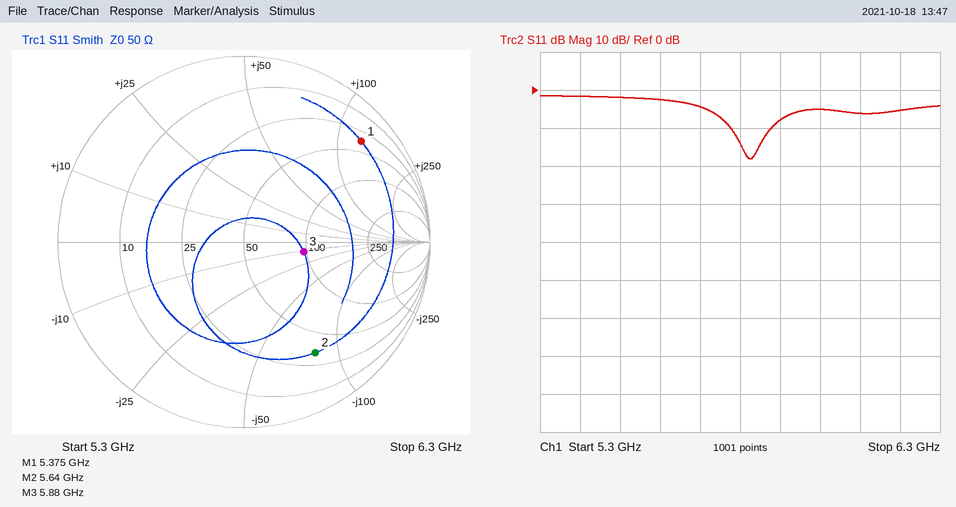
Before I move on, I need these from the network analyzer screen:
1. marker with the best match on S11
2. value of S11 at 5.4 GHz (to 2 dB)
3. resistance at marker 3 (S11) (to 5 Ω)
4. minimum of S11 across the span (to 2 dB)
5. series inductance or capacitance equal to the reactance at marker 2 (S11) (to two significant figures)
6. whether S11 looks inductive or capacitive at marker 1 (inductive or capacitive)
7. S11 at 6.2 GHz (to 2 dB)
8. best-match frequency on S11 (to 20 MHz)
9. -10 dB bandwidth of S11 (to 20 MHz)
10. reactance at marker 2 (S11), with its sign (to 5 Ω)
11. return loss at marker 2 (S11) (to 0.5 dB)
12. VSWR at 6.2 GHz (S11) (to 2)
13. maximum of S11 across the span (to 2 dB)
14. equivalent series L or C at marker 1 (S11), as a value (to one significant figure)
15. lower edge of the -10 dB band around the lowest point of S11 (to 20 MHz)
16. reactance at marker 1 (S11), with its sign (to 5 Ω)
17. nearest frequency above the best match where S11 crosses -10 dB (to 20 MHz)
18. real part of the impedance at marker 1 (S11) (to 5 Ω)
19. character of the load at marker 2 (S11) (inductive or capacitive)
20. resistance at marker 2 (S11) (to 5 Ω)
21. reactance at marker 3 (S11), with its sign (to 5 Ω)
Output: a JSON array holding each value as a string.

["marker 3", "-2 dB", "95 Ω", "-18 dB", "350 fF", "inductive", "-6 dB", "5.82 GHz", "100 MHz", "-80 Ω", "3.0 dB", "4", "-2 dB", "4 nH", "5.78 GHz", "+125 Ω", "5.88 GHz", "35 Ω", "capacitive", "35 Ω", "-10 Ω"]
